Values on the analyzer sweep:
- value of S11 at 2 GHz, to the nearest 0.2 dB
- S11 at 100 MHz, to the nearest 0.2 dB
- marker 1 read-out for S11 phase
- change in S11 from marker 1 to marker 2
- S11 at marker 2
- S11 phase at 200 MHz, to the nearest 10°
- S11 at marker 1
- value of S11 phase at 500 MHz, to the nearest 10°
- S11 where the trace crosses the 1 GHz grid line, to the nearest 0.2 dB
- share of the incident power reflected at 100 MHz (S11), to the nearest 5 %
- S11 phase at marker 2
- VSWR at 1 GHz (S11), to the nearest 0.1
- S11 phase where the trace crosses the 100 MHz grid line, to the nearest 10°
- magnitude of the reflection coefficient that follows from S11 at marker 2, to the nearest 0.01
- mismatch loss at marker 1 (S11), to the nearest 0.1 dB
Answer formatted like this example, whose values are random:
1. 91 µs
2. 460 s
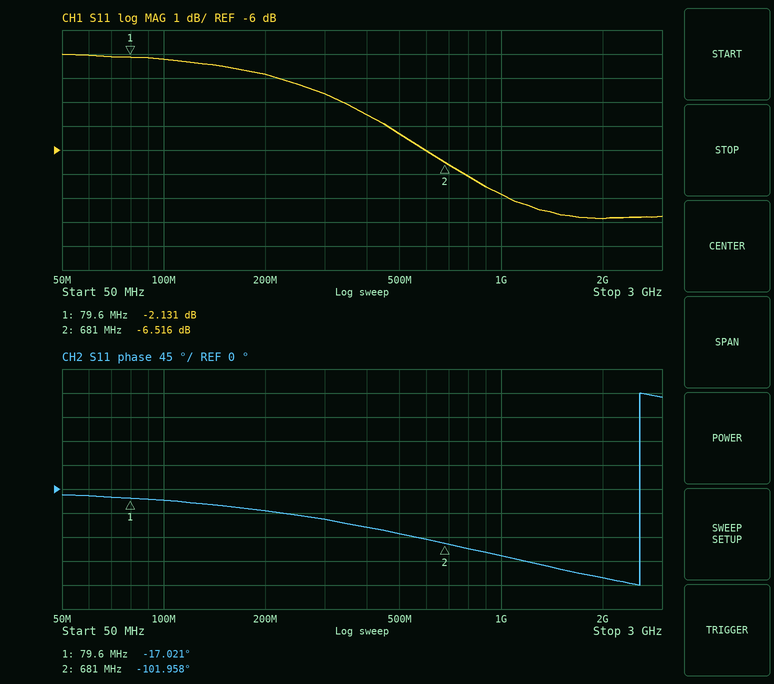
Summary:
1. -8.8 dB
2. -2.2 dB
3. -17.021°
4. -4.385 dB
5. -6.516 dB
6. -40°
7. -2.131 dB
8. -80°
9. -7.8 dB
10. 60 %
11. -101.958°
12. 2.4
13. -20°
14. 0.47
15. 4.1 dB
